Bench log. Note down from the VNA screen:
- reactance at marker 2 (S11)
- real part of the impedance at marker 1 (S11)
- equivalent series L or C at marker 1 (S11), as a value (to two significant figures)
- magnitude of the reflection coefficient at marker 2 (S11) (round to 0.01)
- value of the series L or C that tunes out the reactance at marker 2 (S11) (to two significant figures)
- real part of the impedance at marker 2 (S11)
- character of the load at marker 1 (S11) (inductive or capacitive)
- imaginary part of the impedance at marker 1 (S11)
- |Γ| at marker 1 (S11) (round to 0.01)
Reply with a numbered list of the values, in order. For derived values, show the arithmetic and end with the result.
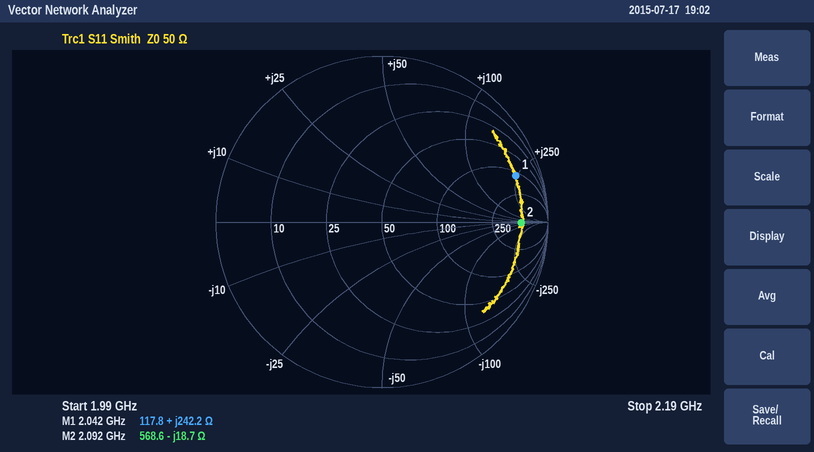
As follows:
1. -18.7 Ω
2. 117.8 Ω
3. L = 242.2 Ω/(2π × 2.042 GHz) ≈ 19 nH
4. 0.84
5. L = 18.7 Ω/(2π × 2.092 GHz) ≈ 1.4 nH
6. 568.6 Ω
7. inductive
8. +242.2 Ω
9. 0.85
